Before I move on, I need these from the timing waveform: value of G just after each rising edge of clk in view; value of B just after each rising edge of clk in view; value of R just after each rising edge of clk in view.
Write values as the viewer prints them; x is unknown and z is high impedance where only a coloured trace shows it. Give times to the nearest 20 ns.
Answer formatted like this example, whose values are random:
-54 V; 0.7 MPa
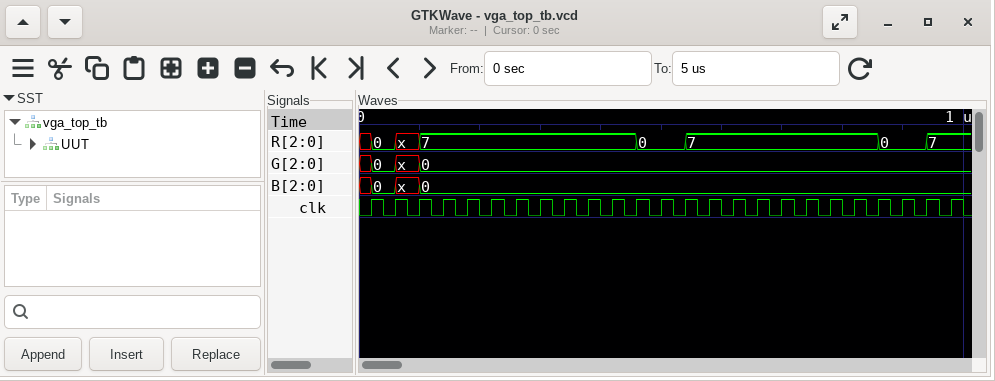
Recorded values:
0, x, 0, 0, 0, 0, 0, 0, 0, 0, 0, 0, 0, 0, 0, 0, 0, 0, 0, 0, 0, 0, 0, 0, 0; 0, x, 0, 0, 0, 0, 0, 0, 0, 0, 0, 0, 0, 0, 0, 0, 0, 0, 0, 0, 0, 0, 0, 0, 0; 0, x, 7, 7, 7, 7, 7, 7, 7, 7, 7, 0, 0, 7, 7, 7, 7, 7, 7, 7, 7, 0, 0, 7, 7
